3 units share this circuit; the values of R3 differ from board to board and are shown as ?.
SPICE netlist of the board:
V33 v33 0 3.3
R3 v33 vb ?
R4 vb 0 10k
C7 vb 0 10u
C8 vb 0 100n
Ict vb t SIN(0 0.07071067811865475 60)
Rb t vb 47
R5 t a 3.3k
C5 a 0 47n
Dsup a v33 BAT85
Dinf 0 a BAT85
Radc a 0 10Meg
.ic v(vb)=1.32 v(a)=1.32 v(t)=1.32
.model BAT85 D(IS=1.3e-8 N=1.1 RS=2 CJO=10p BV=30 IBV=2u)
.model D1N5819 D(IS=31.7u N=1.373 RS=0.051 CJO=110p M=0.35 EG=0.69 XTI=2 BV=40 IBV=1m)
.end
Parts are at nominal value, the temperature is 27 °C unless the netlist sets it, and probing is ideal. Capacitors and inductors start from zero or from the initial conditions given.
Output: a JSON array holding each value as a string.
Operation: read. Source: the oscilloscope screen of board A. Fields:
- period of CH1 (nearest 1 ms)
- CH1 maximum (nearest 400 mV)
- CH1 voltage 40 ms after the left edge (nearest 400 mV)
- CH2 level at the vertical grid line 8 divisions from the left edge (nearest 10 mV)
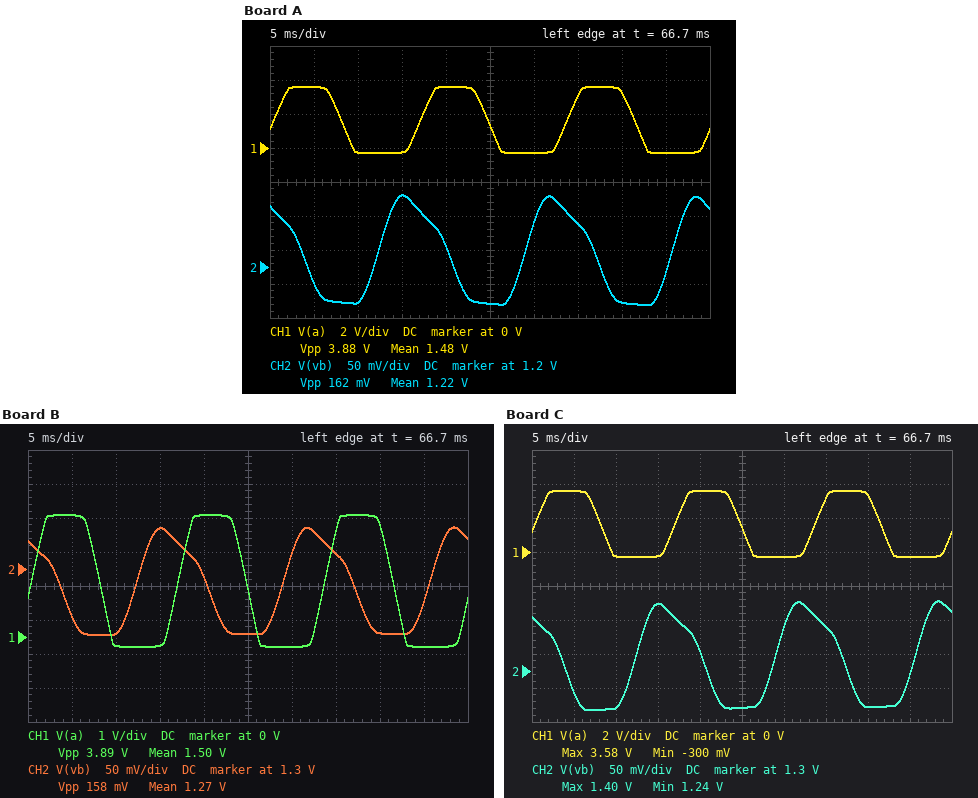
["17 ms", "3.6 V", "3.2 V", "1.15 V"]
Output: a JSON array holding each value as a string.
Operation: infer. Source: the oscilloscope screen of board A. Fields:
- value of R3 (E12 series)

["47 kΩ"]
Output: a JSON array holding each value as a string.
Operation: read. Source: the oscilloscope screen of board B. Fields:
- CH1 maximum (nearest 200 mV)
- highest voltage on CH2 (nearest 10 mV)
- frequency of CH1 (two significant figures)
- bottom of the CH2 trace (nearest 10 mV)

["3.6 V", "1.36 V", "60 Hz", "1.20 V"]
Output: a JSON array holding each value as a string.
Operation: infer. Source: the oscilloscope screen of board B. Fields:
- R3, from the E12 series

["33 kΩ"]
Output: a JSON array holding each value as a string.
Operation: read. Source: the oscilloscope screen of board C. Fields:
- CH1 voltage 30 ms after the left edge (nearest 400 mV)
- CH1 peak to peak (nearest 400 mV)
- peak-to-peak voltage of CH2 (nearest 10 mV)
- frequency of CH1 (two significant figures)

["-400 mV", "4.0 V", "160 mV", "60 Hz"]
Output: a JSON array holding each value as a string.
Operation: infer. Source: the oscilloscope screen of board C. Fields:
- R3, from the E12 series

["27 kΩ"]
